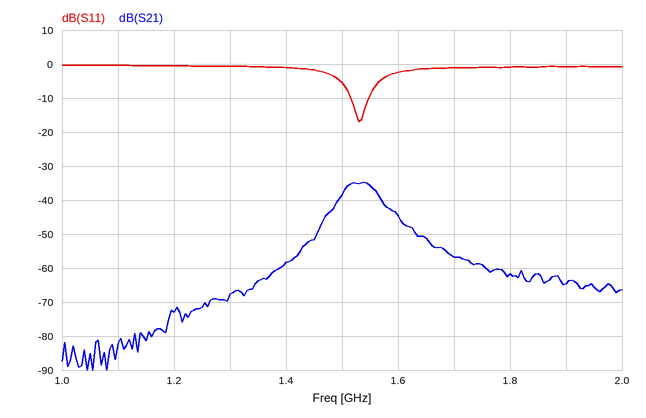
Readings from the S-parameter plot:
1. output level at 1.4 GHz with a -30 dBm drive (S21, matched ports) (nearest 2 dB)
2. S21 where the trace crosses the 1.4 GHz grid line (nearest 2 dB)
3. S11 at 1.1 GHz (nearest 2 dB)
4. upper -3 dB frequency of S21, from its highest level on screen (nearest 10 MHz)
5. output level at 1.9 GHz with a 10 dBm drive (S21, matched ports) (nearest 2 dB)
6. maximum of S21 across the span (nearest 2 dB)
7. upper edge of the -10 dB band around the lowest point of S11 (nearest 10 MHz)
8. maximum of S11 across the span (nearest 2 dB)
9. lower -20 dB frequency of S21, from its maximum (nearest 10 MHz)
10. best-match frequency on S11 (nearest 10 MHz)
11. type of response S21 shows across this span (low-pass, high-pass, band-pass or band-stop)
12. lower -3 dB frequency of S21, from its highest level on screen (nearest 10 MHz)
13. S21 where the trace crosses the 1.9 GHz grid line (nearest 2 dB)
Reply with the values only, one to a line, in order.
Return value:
-88 dBm
-58 dB
0 dB
1.56 GHz
-54 dBm
-34 dB
1.55 GHz
0 dB
1.43 GHz
1.53 GHz
band-pass
1.50 GHz
-64 dB
